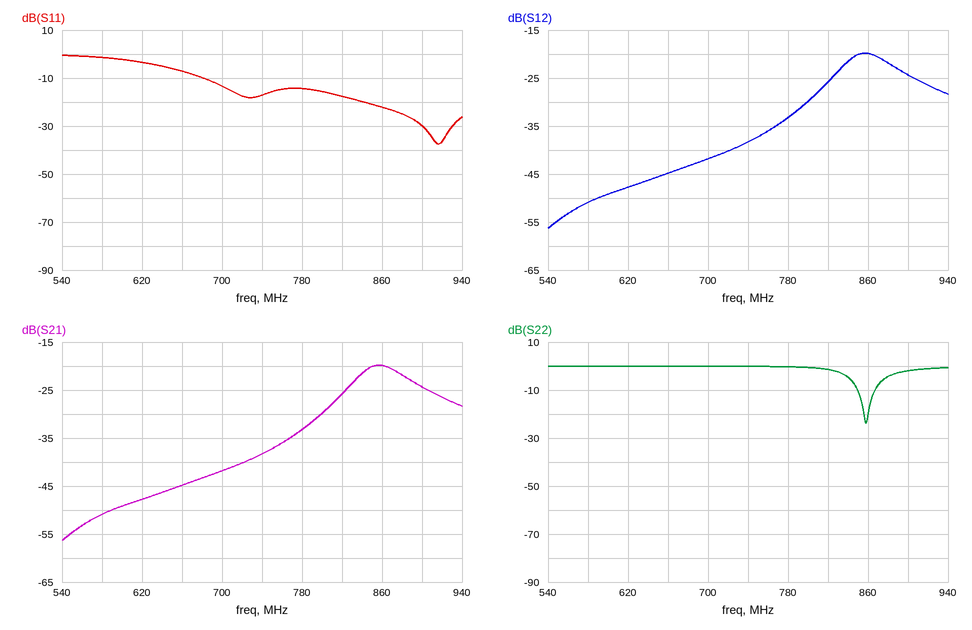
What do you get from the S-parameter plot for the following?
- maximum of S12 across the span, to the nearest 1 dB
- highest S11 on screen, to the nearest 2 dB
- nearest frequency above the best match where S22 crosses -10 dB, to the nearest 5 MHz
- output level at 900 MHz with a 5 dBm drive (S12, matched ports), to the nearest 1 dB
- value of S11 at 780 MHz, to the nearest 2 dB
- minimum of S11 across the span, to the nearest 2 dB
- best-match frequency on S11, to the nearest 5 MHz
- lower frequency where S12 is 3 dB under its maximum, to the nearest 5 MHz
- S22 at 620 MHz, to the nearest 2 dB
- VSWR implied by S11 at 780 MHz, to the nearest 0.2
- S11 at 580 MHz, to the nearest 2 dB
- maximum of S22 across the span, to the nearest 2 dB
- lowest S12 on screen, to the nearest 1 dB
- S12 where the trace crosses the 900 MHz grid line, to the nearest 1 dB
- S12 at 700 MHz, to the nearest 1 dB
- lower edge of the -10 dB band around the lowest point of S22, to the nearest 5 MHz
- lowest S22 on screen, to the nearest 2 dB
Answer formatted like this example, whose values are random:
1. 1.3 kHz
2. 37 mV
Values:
1. -20 dB
2. 0 dB
3. 865 MHz
4. -19 dBm
5. -14 dB
6. -38 dB
7. 915 MHz
8. 835 MHz
9. 0 dB
10. 1.4
11. -2 dB
12. 0 dB
13. -56 dB
14. -24 dB
15. -42 dB
16. 850 MHz
17. -24 dB
